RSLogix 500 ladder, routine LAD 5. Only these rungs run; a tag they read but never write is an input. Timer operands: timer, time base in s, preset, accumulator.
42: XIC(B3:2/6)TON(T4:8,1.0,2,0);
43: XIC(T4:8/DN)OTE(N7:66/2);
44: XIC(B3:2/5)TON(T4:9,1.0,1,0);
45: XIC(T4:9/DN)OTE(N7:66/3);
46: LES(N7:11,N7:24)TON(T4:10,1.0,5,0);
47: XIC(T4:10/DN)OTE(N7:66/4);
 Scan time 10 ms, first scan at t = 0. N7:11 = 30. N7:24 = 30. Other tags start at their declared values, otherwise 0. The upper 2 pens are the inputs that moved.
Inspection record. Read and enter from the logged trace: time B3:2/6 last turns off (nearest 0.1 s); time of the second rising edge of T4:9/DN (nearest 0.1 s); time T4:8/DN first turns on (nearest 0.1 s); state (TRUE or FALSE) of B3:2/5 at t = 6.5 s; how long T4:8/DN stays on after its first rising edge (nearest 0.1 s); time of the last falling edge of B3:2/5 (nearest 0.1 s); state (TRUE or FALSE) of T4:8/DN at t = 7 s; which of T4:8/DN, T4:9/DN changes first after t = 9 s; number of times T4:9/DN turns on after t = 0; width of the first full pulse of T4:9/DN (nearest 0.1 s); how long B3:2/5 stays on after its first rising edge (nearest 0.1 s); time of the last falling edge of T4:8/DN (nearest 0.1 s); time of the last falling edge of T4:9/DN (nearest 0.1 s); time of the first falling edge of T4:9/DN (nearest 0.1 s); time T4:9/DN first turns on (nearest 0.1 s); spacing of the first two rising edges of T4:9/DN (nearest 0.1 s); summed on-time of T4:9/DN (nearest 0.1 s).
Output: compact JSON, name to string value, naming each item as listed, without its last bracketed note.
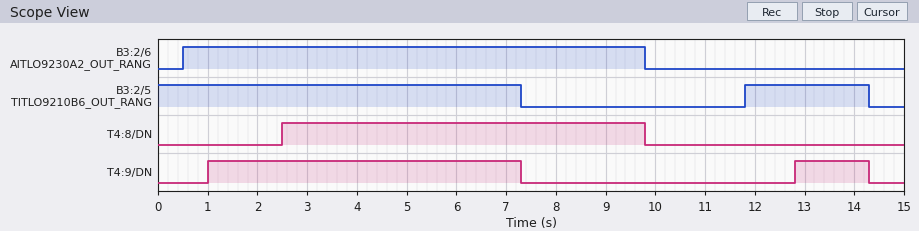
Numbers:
{"time B3:2/6 last turns off": "9.8 s", "time of the second rising edge of T4:9/DN": "12.8 s", "time T4:8/DN first turns on": "2.5 s", "state (TRUE or FALSE) of B3:2/5 at t = 6.5 s": "TRUE", "how long T4:8/DN stays on after its first rising edge": "7.3 s", "time of the last falling edge of B3:2/5": "14.3 s", "state (TRUE or FALSE) of T4:8/DN at t = 7 s": "TRUE", "which of T4:8/DN, T4:9/DN changes first after t = 9 s": "T4:8/DN", "number of times T4:9/DN turns on after t = 0": "2", "width of the first full pulse of T4:9/DN": "6.3 s", "how long B3:2/5 stays on after its first rising edge": "2.5 s", "time of the last falling edge of T4:8/DN": "9.8 s", "time of the last falling edge of T4:9/DN": "14.3 s", "time of the first falling edge of T4:9/DN": "7.3 s", "time T4:9/DN first turns on": "1.0 s", "spacing of the first two rising edges of T4:9/DN": "11.8 s", "summed on-time of T4:9/DN": "7.8 s"}
